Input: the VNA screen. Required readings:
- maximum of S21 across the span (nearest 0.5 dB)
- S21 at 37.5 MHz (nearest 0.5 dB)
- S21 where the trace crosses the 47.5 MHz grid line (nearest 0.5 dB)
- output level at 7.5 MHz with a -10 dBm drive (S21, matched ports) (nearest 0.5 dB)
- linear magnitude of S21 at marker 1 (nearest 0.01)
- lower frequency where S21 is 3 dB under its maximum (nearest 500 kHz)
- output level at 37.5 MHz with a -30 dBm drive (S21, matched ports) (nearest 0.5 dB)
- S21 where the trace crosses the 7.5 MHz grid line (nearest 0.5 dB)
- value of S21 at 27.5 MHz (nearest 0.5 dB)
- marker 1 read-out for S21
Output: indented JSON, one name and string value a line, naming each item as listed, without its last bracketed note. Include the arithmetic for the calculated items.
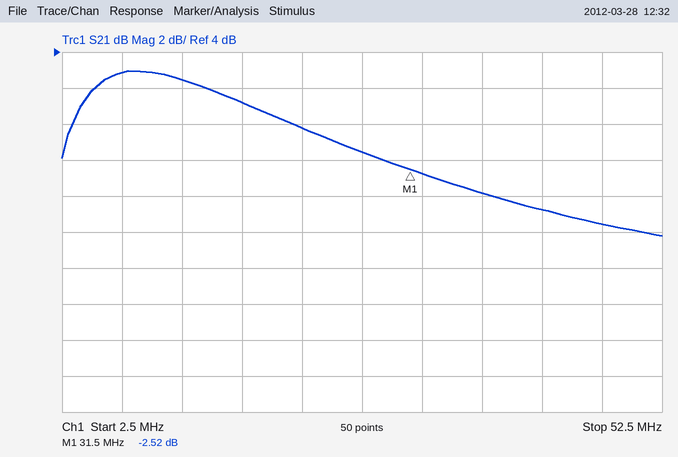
{
  "maximum of S21 across the span": "3.0 dB",
  "S21 at 37.5 MHz": "-4.0 dB",
  "S21 where the trace crosses the 47.5 MHz grid line": "-5.5 dB",
  "output level at 7.5 MHz with a -10 dBm drive (S21, matched ports)": "-10 dBm + (3.0 dB) = -7.0 dBm",
  "linear magnitude of S21 at marker 1": "10^(-2.52/20) ≈ 0.75",
  "lower frequency where S21 is 3 dB under its maximum": "3.5 MHz",
  "output level at 37.5 MHz with a -30 dBm drive (S21, matched ports)": "-30 dBm + (-4.0 dB) = -34.0 dBm",
  "S21 where the trace crosses the 7.5 MHz grid line": "3.0 dB",
  "value of S21 at 27.5 MHz": "-1.5 dB",
  "marker 1 read-out for S21": "-2.52 dB"
}
